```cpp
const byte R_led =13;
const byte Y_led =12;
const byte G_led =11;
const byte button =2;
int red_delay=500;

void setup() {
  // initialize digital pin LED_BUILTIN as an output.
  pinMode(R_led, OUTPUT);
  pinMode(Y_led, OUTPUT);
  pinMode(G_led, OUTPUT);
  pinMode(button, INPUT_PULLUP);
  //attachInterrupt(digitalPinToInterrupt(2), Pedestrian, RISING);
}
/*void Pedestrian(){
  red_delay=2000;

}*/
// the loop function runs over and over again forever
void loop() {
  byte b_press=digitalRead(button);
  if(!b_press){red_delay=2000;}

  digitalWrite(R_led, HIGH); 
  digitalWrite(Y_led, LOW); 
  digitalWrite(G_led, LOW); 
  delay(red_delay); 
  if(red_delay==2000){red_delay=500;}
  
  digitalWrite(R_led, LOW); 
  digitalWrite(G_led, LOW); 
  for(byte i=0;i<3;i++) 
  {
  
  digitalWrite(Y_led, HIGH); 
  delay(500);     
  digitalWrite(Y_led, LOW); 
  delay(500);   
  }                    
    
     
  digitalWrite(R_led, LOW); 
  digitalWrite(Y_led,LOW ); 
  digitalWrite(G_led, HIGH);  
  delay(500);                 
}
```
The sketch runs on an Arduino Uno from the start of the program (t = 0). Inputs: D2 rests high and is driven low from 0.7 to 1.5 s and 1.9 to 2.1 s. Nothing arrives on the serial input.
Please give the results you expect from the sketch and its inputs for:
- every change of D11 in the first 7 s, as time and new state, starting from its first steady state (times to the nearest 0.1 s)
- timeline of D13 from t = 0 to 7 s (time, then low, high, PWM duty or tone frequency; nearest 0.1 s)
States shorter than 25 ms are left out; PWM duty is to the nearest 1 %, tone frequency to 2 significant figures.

0 s low; 3.5 s high; 4 s low
0 s high; 0.5 s low; 4 s high; 4.5 s low
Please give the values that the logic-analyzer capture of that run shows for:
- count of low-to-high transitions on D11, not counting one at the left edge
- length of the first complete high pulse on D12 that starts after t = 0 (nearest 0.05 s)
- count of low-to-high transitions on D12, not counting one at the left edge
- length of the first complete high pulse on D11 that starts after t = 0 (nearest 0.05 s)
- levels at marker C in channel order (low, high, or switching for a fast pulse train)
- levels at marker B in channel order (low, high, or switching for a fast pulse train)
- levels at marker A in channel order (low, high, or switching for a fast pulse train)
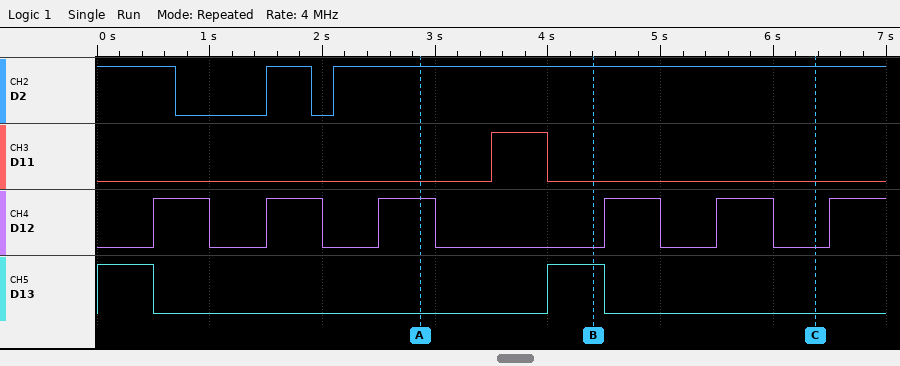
1
0.50 s
6
0.50 s
D2 high, D11 low, D12 low, D13 low
D2 high, D11 low, D12 low, D13 high
D2 high, D11 low, D12 high, D13 low
